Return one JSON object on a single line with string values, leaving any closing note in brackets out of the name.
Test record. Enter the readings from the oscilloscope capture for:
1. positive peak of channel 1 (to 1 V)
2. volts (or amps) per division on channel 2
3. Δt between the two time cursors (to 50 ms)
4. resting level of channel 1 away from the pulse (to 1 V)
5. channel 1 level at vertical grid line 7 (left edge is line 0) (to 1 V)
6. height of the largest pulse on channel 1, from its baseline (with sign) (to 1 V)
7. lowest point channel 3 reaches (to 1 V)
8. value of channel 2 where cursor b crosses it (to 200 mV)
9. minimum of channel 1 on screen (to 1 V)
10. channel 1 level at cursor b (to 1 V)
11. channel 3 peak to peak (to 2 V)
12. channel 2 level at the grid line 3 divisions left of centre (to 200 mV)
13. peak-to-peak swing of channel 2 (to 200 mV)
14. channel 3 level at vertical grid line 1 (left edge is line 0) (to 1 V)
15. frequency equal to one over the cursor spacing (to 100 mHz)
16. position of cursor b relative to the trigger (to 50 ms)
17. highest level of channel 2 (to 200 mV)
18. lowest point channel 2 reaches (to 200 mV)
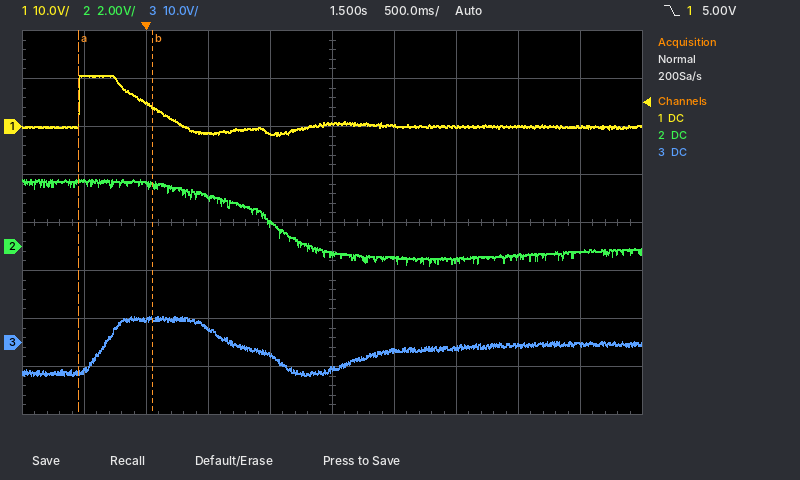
{"positive peak of channel 1": "11 V", "volts (or amps) per division on channel 2": "2 V", "Δt between the two time cursors": "600 ms", "resting level of channel 1 away from the pulse": "0 V", "channel 1 level at vertical grid line 7 (left edge is line 0)": "0 V", "height of the largest pulse on channel 1, from its baseline (with sign)": "+11 V", "lowest point channel 3 reaches": "-7 V", "value of channel 2 where cursor b crosses it": "2.6 V", "minimum of channel 1 on screen": "-2 V", "channel 1 level at cursor b": "4 V", "channel 3 peak to peak": "12 V", "channel 2 level at the grid line 3 divisions left of centre": "2.6 V", "peak-to-peak swing of channel 2": "3.6 V", "channel 3 level at vertical grid line 1 (left edge is line 0)": "-6 V", "frequency equal to one over the cursor spacing": "1.7 Hz", "position of cursor b relative to the trigger": "+50 ms", "highest level of channel 2": "2.8 V", "lowest point channel 2 reaches": "-800 mV"}
